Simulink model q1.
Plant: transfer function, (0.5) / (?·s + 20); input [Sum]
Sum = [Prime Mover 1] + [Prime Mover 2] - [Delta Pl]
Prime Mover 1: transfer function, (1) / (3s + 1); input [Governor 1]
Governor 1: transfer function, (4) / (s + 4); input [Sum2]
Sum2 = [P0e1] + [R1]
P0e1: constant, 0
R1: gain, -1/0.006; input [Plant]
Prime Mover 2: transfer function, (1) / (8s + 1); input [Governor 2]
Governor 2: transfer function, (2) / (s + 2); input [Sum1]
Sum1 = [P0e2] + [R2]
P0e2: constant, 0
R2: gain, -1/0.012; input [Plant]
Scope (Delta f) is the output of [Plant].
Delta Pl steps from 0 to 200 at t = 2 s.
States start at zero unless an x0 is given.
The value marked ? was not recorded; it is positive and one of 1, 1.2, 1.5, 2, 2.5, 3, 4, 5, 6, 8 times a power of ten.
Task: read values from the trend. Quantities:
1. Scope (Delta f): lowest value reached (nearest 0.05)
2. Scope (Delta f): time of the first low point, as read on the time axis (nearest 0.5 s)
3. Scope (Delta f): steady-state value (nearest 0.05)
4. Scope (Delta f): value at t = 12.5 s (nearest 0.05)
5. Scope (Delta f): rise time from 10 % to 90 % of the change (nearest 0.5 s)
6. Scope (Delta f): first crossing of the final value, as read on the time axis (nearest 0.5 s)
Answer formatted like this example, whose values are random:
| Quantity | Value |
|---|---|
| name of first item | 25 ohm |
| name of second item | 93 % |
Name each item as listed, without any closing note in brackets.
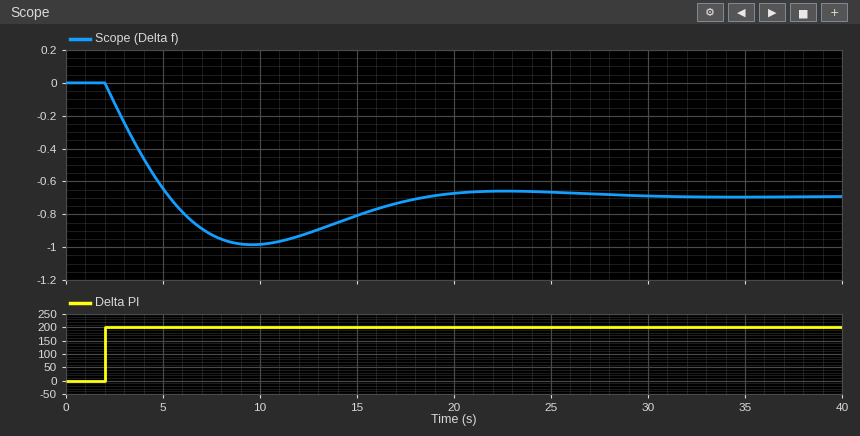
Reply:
| Quantity | Value |
|---|---|
| Scope (Delta f): lowest value reached | -1.00 |
| Scope (Delta f): time of the first low point, as read on the time axis | 9.5 s |
| Scope (Delta f): steady-state value | -0.70 |
| Scope (Delta f): value at t = 12.5 s | -0.90 |
| Scope (Delta f): rise time from 10 % to 90 % of the change | 2.5 s |
| Scope (Delta f): first crossing of the final value, as read on the time axis | 5.5 s |
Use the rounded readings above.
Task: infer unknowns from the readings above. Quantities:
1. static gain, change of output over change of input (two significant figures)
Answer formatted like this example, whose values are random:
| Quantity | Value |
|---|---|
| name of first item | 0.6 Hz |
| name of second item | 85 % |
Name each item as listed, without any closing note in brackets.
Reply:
| Quantity | Value |
|---|---|
| static gain, change of output over change of input | -0.0035 |
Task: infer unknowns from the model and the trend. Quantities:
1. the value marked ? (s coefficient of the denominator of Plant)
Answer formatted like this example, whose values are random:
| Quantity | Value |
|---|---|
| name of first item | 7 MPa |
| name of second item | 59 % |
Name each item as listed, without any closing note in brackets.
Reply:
| Quantity | Value |
|---|---|
| the value marked ? | 400 |
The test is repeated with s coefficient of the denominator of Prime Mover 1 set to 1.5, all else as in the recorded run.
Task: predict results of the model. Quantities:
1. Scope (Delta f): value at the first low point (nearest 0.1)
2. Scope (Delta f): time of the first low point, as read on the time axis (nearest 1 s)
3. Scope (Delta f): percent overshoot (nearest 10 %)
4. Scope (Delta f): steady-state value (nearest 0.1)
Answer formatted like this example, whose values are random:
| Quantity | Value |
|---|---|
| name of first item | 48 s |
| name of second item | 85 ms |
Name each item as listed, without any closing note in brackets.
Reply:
| Quantity | Value |
|---|---|
| Scope (Delta f): value at the first low point | -0.9 |
| Scope (Delta f): time of the first low point, as read on the time axis | 9 s |
| Scope (Delta f): percent overshoot | 30 % |
| Scope (Delta f): steady-state value | -0.7 |
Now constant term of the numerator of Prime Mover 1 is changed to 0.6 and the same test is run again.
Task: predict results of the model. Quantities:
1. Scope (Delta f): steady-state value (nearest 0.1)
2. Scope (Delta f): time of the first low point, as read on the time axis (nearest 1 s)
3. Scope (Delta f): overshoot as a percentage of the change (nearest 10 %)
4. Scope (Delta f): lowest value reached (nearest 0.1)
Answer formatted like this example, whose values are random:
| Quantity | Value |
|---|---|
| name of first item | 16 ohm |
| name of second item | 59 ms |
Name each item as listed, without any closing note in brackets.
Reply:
| Quantity | Value |
|---|---|
| Scope (Delta f): steady-state value | -0.9 |
| Scope (Delta f): time of the first low point, as read on the time axis | 12 s |
| Scope (Delta f): overshoot as a percentage of the change | 30 % |
| Scope (Delta f): lowest value reached | -1.2 |
